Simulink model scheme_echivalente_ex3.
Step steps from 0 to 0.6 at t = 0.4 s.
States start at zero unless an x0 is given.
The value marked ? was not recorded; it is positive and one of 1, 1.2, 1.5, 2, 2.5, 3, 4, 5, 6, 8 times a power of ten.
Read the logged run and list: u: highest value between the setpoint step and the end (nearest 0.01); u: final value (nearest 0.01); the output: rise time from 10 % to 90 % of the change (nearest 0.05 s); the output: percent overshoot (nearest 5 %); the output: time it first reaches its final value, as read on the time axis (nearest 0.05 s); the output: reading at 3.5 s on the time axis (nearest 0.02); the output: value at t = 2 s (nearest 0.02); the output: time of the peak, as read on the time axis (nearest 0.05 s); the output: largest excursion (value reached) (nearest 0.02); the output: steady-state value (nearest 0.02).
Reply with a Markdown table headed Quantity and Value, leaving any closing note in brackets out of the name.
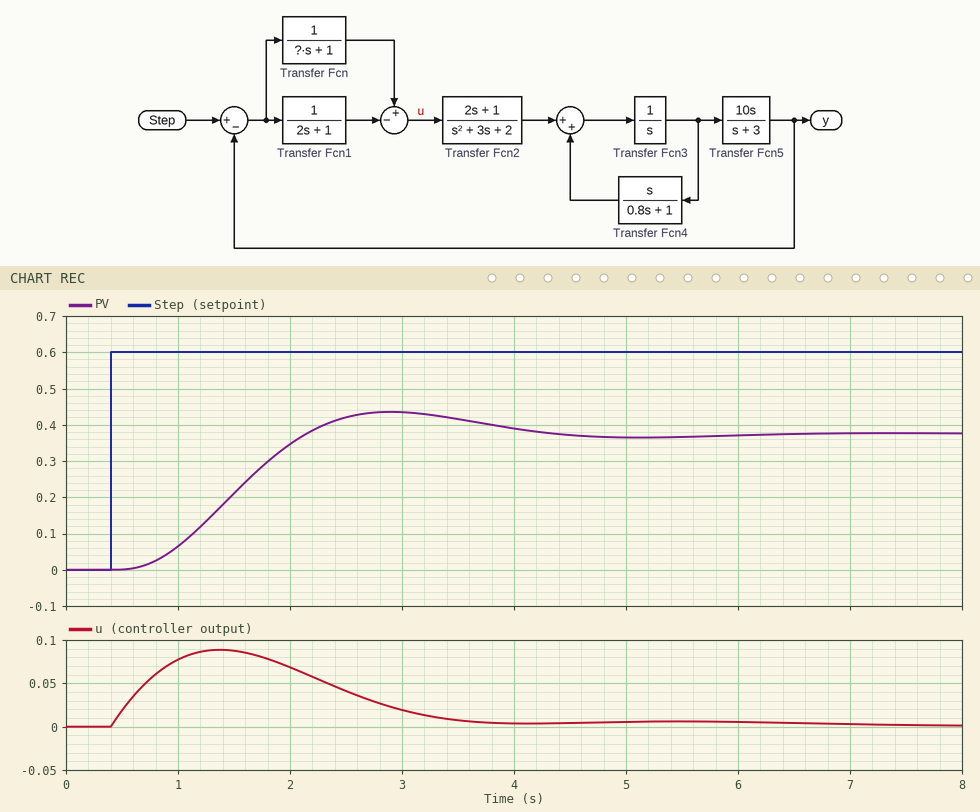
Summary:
| Quantity | Value |
|---|---|
| u: highest value between the setpoint step and the end | 0.09 |
| u: final value | 0.00 |
| the output: rise time from 10 % to 90 % of the change | 1.10 s |
| the output: percent overshoot | 15 % |
| the output: time it first reaches its final value, as read on the time axis | 2.15 s |
| the output: reading at 3.5 s on the time axis | 0.42 |
| the output: value at t = 2 s | 0.34 |
| the output: time of the peak, as read on the time axis | 2.90 s |
| the output: largest excursion (value reached) | 0.44 |
| the output: steady-state value | 0.38 |
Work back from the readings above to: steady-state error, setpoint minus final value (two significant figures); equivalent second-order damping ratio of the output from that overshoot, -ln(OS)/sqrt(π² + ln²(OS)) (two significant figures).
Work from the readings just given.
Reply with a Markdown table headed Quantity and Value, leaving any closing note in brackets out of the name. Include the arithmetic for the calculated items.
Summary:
| Quantity | Value |
|---|---|
| steady-state error, setpoint minus final value | 0.6 - 0.38 = 0.22 |
| equivalent second-order damping ratio of the output from that overshoot, -ln(OS)/sqrt(π² + ln²(OS)) | ln(0.15) = -1.897; 1.897 / sqrt(9.870 + 3.599) = 0.52 |
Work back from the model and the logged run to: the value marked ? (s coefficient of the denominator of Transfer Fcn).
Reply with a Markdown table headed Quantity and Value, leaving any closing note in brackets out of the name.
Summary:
| Quantity | Value |
|---|---|
| the value marked ? | 1.2 |
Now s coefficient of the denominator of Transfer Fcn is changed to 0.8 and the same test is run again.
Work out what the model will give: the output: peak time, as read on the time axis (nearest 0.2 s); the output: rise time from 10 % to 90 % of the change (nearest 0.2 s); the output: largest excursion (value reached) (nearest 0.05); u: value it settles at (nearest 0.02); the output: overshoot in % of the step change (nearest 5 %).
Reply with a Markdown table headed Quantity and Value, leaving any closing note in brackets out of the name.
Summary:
| Quantity | Value |
|---|---|
| the output: peak time, as read on the time axis | 2.2 s |
| the output: rise time from 10 % to 90 % of the change | 0.8 s |
| the output: largest excursion (value reached) | 0.55 |
| u: value it settles at | 0.00 |
| the output: overshoot in % of the step change | 30 % |
